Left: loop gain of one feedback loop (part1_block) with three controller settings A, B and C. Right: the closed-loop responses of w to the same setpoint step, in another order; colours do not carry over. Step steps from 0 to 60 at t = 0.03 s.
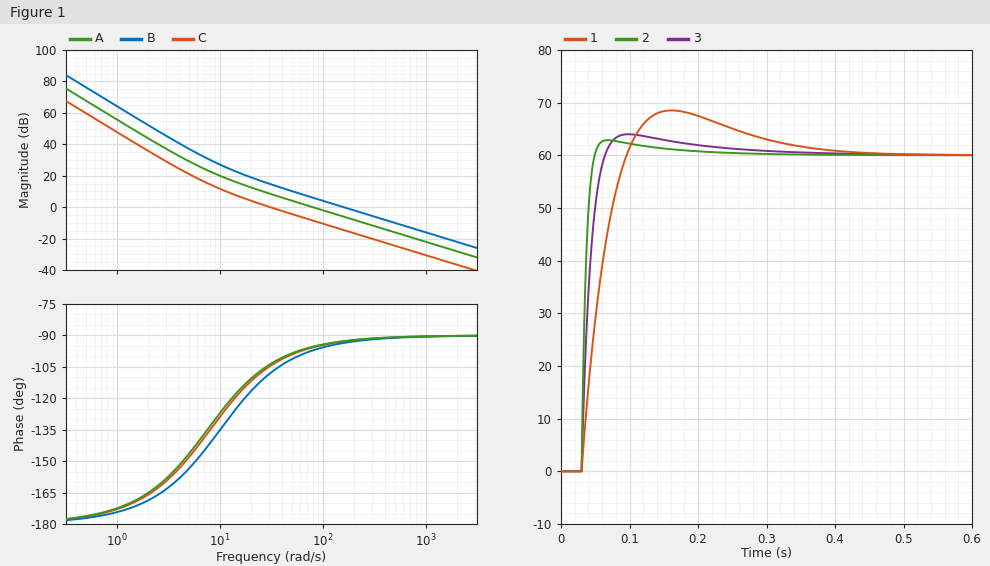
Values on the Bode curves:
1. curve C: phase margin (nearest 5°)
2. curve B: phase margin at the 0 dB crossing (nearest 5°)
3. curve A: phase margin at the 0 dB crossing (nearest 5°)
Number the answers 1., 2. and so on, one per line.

1. 75°
2. 85°
3. 85°
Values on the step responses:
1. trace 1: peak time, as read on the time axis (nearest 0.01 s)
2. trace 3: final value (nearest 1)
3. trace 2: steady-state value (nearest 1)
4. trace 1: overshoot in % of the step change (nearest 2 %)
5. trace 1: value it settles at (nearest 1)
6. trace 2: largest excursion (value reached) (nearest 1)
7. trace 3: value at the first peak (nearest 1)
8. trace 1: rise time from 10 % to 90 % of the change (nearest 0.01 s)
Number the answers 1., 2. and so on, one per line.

1. 0.16 s
2. 60
3. 60
4. 14 %
5. 60
6. 63
7. 64
8. 0.05 s
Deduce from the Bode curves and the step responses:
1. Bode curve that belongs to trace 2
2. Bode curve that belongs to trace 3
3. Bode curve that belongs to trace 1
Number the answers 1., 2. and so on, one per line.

1. B
2. A
3. C
